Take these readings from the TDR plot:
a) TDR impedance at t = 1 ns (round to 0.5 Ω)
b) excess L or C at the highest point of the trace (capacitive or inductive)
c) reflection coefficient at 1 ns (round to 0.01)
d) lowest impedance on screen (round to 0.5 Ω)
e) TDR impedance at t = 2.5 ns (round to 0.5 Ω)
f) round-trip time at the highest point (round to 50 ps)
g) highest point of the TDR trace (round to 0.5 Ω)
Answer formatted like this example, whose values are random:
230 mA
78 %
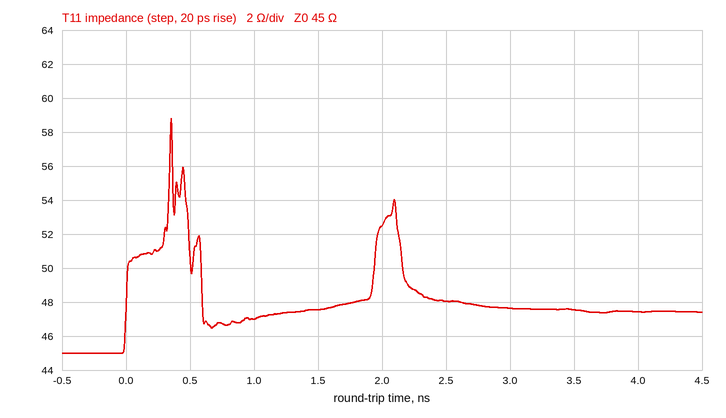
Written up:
47.0 Ω
inductive
+0.02
45.0 Ω
48.0 Ω
350 ps
59.0 Ω
